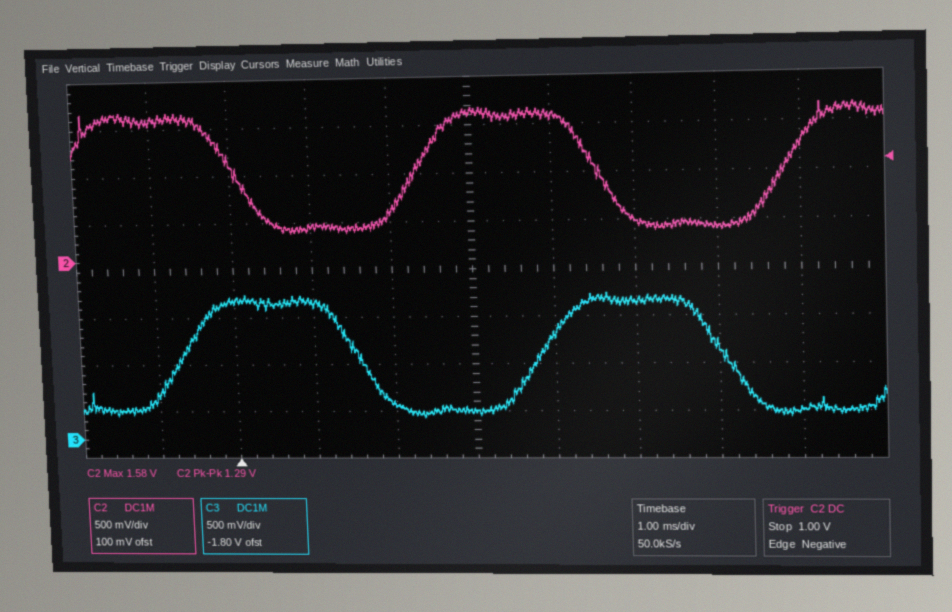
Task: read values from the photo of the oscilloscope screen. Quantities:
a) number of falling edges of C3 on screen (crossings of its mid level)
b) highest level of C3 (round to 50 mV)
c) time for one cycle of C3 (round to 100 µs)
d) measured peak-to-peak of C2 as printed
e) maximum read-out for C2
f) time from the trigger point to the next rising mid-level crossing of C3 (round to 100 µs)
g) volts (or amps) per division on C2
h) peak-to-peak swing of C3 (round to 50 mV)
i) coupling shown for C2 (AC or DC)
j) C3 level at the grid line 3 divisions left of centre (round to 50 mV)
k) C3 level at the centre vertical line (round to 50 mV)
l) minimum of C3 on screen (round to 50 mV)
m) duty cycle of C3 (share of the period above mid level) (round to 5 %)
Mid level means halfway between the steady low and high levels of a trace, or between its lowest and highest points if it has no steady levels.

2
1.55 V
4.5 ms
1.29 V
1.58 V
3.8 ms
500 mV
1.30 V
DC
1.50 V
300 mV
250 mV
50 %
